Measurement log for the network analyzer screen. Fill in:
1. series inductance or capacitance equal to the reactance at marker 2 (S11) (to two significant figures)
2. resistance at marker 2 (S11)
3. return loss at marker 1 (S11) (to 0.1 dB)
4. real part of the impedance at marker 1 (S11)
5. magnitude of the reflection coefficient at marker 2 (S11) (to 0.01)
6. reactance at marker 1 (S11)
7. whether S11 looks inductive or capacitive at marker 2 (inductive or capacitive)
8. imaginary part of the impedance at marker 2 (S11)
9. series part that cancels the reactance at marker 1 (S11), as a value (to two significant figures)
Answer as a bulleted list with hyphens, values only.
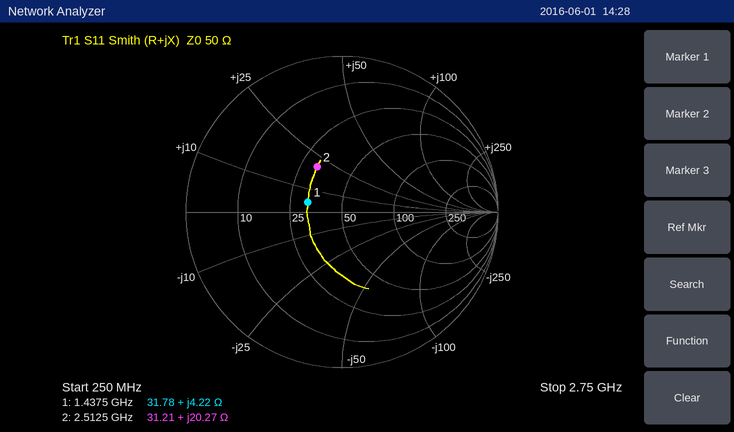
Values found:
- 1.3 nH
- 31.21 Ω
- 12.8 dB
- 31.78 Ω
- 0.33
- +4.22 Ω
- inductive
- +20.27 Ω
- 26 pF
